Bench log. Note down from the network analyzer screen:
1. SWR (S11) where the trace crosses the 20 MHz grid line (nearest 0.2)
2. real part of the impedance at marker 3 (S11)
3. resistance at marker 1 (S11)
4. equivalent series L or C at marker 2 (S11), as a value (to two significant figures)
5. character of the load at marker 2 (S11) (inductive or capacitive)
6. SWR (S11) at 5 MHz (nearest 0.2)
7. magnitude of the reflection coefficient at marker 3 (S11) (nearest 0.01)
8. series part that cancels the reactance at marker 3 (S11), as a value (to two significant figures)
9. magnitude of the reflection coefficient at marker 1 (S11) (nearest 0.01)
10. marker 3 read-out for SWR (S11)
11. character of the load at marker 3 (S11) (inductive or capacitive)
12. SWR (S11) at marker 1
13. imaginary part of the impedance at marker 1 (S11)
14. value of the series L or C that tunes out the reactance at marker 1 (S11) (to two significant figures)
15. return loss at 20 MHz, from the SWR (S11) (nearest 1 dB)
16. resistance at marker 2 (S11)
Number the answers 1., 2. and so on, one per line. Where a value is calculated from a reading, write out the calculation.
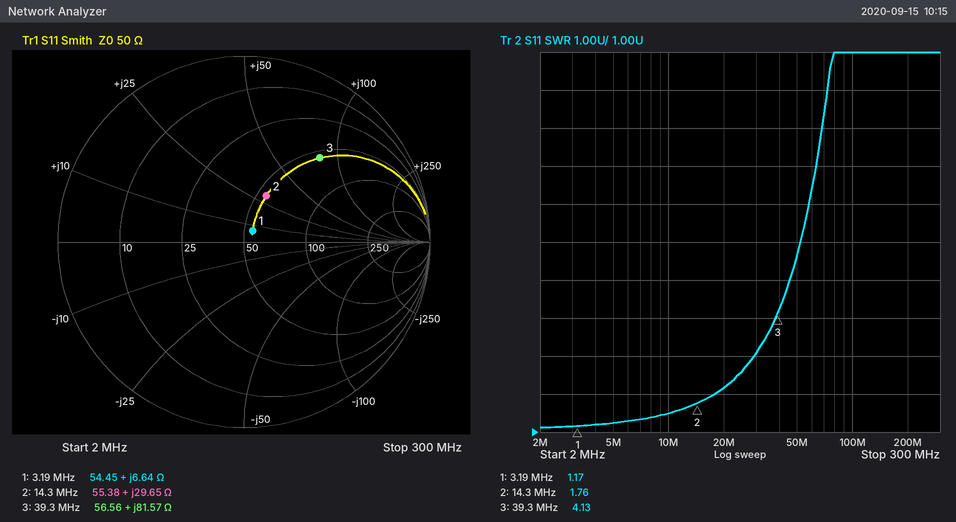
1. 2.2
2. 56.56 Ω
3. 54.45 Ω
4. L = 29.65 Ω/(2π × 14.3 MHz) ≈ 330 nH
5. inductive
6. 1.2
7. 0.61
8. C = 1/(2π × 39.3 MHz × 81.57 Ω) ≈ 50 pF
9. 0.08
10. 4.13
11. inductive
12. 1.17
13. +6.64 Ω
14. C = 1/(2π × 3.19 MHz × 6.64 Ω) ≈ 7.5 nF
15. −20 log10((2.2 − 1)/(2.2 + 1)) ≈ 9 dB
16. 55.38 Ω
